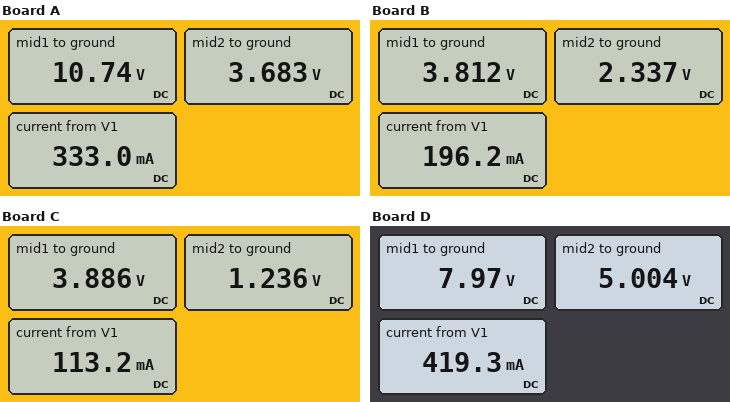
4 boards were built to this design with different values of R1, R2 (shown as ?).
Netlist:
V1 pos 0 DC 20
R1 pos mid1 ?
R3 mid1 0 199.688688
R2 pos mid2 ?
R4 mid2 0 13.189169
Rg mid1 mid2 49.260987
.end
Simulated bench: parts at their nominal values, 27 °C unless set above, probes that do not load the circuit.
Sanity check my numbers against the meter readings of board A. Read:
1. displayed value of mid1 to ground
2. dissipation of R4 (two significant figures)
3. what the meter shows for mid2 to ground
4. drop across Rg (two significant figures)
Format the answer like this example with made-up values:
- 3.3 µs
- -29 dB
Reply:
- 10.74 V
- 1.0 W
- 3.683 V
- 7.1 V
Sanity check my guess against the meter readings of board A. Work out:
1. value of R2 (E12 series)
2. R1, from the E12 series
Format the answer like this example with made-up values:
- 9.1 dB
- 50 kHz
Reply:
- 120 Ω
- 47 Ω
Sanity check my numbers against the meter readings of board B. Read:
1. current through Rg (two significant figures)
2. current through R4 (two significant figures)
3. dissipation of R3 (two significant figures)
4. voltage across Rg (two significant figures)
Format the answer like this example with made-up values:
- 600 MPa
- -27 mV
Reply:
- 30 mA
- 180 mA
- 73 mW
- 1.5 V
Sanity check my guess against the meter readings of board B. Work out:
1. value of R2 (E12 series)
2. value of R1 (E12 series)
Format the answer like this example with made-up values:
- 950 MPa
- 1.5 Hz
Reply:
- 120 Ω
- 330 Ω
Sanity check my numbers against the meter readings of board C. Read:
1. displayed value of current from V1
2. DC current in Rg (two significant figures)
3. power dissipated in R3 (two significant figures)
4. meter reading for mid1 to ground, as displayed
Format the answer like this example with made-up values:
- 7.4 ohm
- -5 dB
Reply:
- 113.2 mA
- 54 mA
- 76 mW
- 3.886 V
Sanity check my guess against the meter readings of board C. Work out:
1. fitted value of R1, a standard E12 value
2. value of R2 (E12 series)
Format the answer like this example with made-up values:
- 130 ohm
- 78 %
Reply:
- 220 Ω
- 470 Ω
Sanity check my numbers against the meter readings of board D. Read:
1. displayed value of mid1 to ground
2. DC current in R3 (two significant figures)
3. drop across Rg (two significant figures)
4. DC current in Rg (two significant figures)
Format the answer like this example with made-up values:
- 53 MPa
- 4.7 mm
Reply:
- 7.97 V
- 40 mA
- 3.0 V
- 60 mA
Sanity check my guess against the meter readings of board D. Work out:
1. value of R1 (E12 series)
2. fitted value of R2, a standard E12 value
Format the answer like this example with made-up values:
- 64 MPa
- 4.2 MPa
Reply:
- 120 Ω
- 47 Ω
